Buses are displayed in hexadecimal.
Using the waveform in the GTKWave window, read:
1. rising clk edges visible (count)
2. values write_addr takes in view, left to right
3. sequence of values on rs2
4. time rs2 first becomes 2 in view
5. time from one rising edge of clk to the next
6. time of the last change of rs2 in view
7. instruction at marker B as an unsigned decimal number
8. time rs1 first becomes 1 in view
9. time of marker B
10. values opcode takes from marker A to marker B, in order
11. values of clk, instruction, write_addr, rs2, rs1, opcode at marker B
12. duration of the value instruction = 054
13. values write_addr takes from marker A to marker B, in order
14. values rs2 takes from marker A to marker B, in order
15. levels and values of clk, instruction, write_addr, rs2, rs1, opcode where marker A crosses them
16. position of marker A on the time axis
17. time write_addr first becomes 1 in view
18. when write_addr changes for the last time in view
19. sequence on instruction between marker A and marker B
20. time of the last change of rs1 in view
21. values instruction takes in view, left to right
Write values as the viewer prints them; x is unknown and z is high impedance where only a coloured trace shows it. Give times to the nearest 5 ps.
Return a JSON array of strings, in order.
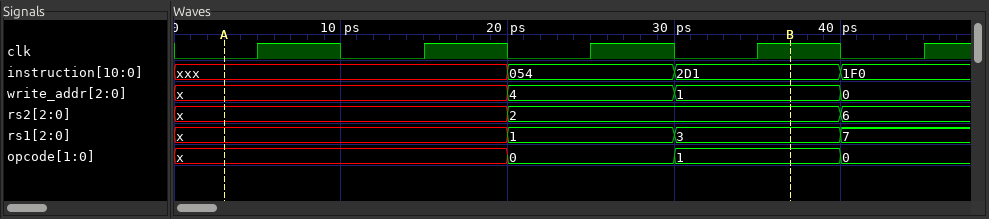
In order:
["5", "x, 4, 1, 0", "x, 2, 6", "20 ps", "10 ps", "40 ps", "721", "20 ps", "35 ps", "x, 0, 1", "clk=1, instruction=2D1, write_addr=1, rs2=2, rs1=3, opcode=1", "10 ps", "x, 4, 1", "x, 2", "clk=0, instruction=xxx, write_addr=x, rs2=x, rs1=x, opcode=x", "5 ps", "30 ps", "40 ps", "xxx, 054, 2D1", "40 ps", "xxx, 054, 2D1, 1F0"]
